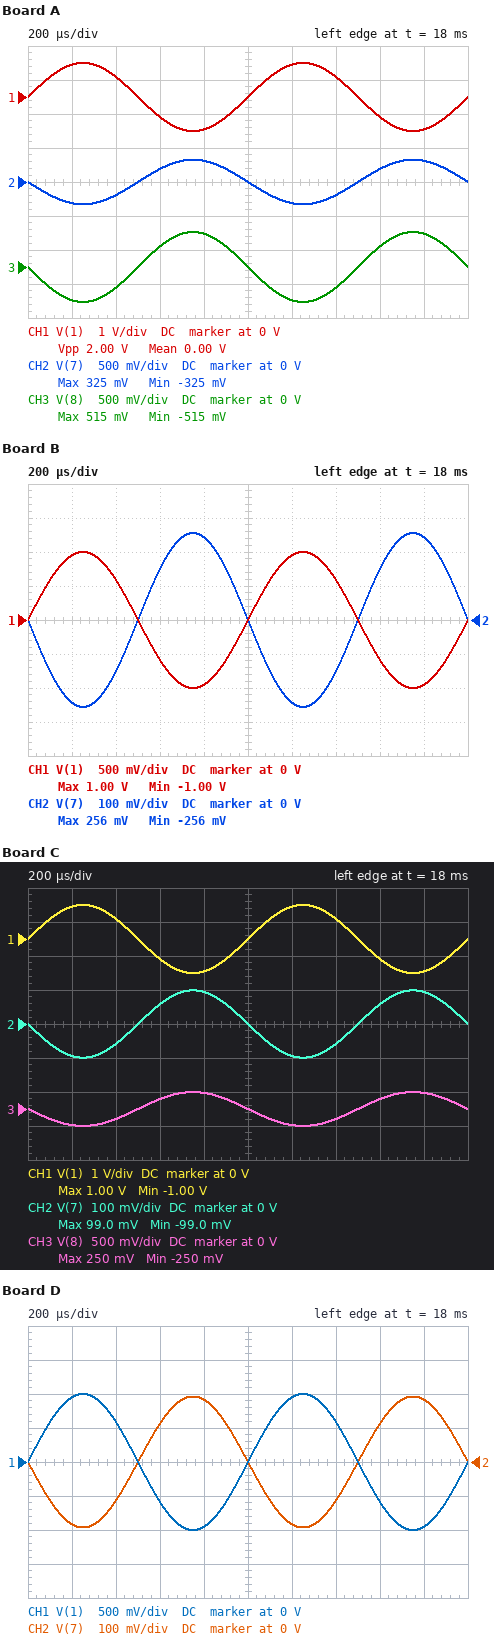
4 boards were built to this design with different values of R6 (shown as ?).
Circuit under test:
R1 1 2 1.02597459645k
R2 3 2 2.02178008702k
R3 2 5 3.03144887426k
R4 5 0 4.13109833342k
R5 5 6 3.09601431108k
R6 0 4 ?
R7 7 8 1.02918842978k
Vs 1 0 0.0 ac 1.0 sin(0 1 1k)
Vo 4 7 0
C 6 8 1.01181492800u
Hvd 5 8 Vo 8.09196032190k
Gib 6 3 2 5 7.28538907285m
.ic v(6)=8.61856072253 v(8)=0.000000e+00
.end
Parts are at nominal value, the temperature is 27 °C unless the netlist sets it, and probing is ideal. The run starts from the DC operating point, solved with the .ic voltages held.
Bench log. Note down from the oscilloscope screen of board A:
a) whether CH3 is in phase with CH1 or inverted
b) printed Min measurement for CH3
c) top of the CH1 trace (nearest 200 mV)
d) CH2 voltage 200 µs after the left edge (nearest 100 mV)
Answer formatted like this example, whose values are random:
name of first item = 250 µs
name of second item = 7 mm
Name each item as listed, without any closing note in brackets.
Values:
whether CH3 is in phase with CH1 or inverted = inverted
printed Min measurement for CH3 = -515 mV
top of the CH1 trace = 1.0 V
CH2 voltage 200 µs after the left edge = -300 mV
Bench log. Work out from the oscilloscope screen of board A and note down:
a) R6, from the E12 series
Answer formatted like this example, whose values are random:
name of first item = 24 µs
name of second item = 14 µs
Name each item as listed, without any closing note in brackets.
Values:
R6, from the E12 series = 1.8 kΩ
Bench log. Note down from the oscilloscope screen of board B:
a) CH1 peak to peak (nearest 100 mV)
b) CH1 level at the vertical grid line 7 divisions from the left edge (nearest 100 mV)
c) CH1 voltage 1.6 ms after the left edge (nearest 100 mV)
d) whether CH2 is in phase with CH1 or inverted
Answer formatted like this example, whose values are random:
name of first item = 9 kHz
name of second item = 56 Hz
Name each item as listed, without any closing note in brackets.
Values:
CH1 peak to peak = 2.0 V
CH1 level at the vertical grid line 7 divisions from the left edge = 600 mV
CH1 voltage 1.6 ms after the left edge = -600 mV
whether CH2 is in phase with CH1 or inverted = inverted
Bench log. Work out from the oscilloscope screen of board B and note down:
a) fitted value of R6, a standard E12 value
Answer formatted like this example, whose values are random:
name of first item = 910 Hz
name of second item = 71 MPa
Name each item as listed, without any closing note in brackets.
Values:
fitted value of R6, a standard E12 value = 1.5 kΩ
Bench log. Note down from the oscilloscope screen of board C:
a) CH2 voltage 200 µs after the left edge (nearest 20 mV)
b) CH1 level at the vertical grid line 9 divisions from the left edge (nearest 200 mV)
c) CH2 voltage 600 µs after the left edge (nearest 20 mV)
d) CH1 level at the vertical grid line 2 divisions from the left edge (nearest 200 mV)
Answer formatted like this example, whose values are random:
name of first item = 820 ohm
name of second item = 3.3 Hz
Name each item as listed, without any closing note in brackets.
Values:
CH2 voltage 200 µs after the left edge = -100 mV
CH1 level at the vertical grid line 9 divisions from the left edge = -1.0 V
CH2 voltage 600 µs after the left edge = 60 mV
CH1 level at the vertical grid line 2 divisions from the left edge = 600 mV
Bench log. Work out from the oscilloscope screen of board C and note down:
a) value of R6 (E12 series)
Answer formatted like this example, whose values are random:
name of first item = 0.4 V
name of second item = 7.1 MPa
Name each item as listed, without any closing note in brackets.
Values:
value of R6 = 680 Ω
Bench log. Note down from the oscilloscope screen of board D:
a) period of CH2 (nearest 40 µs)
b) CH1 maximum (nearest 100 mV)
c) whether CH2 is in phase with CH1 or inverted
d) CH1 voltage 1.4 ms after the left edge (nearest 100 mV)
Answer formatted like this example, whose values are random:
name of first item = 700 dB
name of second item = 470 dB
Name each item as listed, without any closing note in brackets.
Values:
period of CH2 = 1.00 ms
CH1 maximum = 1.0 V
whether CH2 is in phase with CH1 or inverted = inverted
CH1 voltage 1.4 ms after the left edge = 600 mV
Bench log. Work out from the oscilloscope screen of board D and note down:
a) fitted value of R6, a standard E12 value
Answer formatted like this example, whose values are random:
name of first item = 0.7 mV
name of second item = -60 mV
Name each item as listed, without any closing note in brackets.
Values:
fitted value of R6, a standard E12 value = 1.2 kΩ
